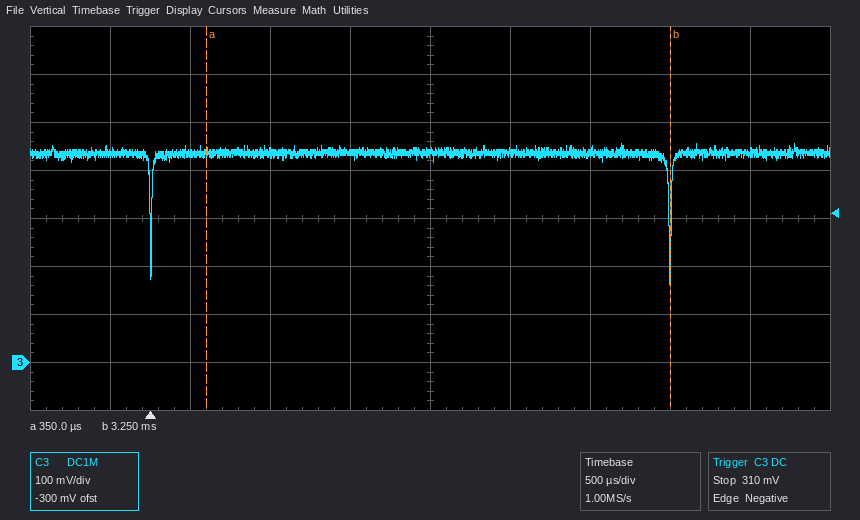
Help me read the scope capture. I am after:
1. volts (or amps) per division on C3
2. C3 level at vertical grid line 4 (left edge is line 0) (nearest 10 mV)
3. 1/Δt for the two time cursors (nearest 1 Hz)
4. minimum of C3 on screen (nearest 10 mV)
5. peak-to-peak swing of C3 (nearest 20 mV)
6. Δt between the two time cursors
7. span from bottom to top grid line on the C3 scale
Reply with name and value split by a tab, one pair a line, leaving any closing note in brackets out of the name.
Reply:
volts (or amps) per division on C3	100 mV
C3 level at vertical grid line 4 (left edge is line 0)	440 mV
1/Δt for the two time cursors	345 Hz
minimum of C3 on screen	160 mV
peak-to-peak swing of C3	300 mV
Δt between the two time cursors	2.90 ms
span from bottom to top grid line on the C3 scale	800 mV
